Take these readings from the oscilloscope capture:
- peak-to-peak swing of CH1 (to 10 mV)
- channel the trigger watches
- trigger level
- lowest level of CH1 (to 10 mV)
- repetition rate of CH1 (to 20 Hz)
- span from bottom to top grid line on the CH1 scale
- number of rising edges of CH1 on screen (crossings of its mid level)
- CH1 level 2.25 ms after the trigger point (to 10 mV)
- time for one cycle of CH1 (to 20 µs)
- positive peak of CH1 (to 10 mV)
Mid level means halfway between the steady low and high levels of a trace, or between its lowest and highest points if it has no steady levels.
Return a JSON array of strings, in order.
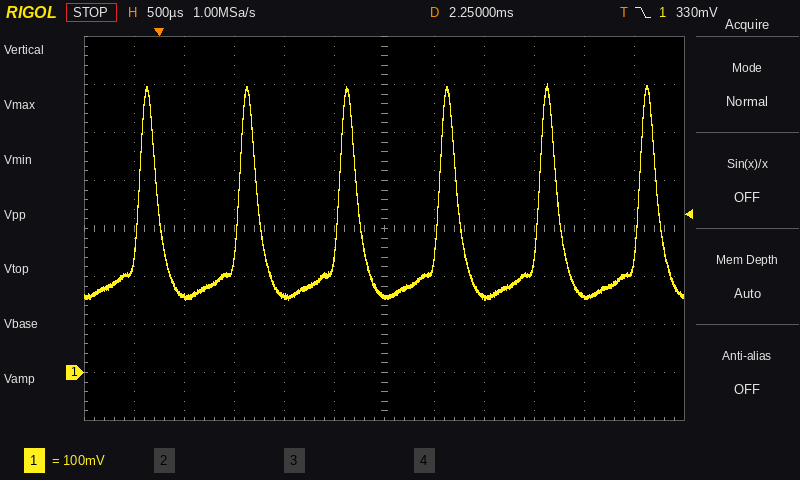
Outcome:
["450 mV", "CH1", "330 mV", "150 mV", "1.00 kHz", "800 mV", "6", "160 mV", "1.00 ms", "600 mV"]
